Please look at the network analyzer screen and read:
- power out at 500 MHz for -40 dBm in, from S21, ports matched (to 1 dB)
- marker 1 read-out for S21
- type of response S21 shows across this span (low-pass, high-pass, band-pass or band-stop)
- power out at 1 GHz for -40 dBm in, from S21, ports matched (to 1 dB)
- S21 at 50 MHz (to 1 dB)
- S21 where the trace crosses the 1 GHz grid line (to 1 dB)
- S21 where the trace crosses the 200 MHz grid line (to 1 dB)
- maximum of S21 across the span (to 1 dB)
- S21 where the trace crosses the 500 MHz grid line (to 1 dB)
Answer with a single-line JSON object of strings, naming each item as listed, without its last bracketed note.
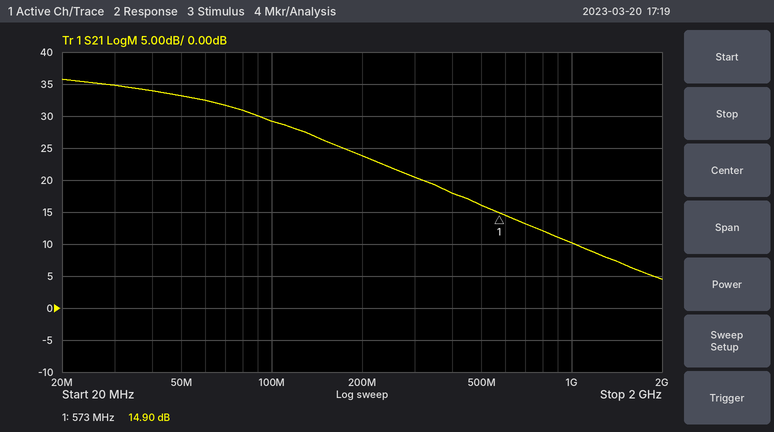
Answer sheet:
{"power out at 500 MHz for -40 dBm in, from S21, ports matched": "-24 dBm", "marker 1 read-out for S21": "14.90 dB", "type of response S21 shows across this span": "low-pass", "power out at 1 GHz for -40 dBm in, from S21, ports matched": "-30 dBm", "S21 at 50 MHz": "33 dB", "S21 where the trace crosses the 1 GHz grid line": "10 dB", "S21 where the trace crosses the 200 MHz grid line": "24 dB", "maximum of S21 across the span": "36 dB", "S21 where the trace crosses the 500 MHz grid line": "16 dB"}
